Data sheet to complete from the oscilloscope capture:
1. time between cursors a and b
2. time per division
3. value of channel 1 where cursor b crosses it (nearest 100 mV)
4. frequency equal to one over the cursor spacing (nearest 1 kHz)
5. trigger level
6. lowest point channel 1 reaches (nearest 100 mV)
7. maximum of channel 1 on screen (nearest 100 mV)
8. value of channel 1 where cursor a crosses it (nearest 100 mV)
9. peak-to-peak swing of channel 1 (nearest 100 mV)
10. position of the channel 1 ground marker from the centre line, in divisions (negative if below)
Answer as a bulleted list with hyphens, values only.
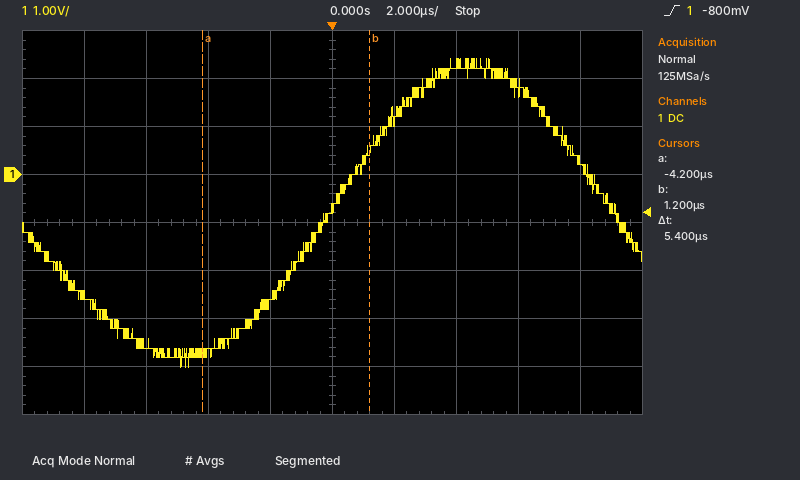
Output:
- 5.4 µs
- 2 µs
- 500 mV
- 185 kHz
- -800 mV
- -4.0 V
- 2.4 V
- -3.7 V
- 6.4 V
- +1.0 div
